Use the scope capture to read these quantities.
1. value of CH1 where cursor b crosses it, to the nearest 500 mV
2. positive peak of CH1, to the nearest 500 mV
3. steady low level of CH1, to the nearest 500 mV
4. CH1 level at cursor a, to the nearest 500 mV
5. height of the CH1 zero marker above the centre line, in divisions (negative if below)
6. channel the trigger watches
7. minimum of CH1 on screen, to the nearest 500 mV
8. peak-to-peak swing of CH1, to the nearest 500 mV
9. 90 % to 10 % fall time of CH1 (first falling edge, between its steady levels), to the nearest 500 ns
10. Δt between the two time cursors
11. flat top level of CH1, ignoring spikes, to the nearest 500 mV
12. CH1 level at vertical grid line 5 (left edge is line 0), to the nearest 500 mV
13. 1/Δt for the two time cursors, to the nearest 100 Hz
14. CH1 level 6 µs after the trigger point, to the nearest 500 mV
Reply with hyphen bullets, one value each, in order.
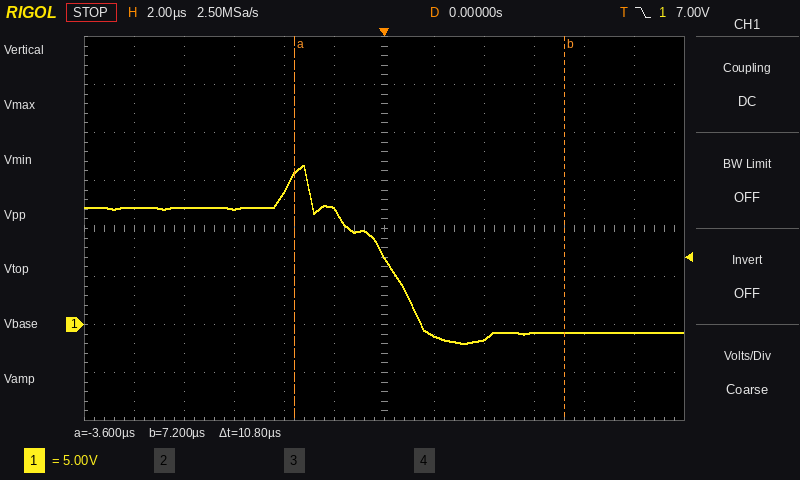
- -1.0 V
- 16.5 V
- -1.0 V
- 15.5 V
- -2.0 div
- CH1
- -2.0 V
- 18.5 V
- 3.0 µs
- 10.8 µs
- 12.0 V
- 12.0 V
- 92.6 kHz
- -1.0 V
